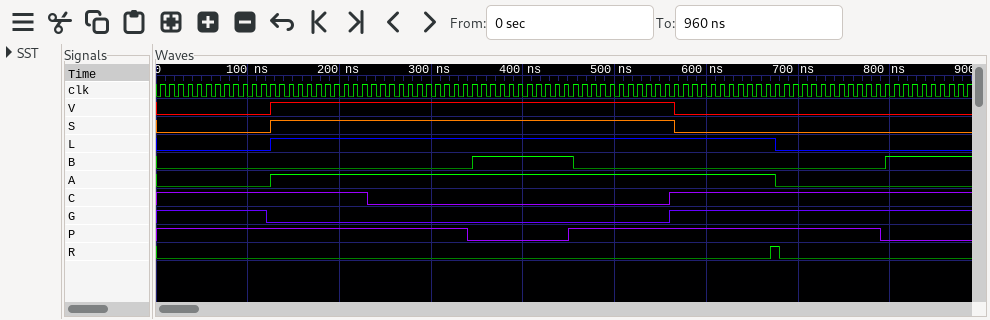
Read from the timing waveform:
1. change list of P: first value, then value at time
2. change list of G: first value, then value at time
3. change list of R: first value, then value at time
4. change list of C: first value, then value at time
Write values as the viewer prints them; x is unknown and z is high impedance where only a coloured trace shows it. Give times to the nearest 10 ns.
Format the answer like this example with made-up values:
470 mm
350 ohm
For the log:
1, 0 at 340 ns, 1 at 450 ns, 0 at 790 ns
1, 0 at 120 ns, 1 at 560 ns
0, 1 at 670 ns, 0 at 680 ns
1, 0 at 230 ns, 1 at 560 ns
